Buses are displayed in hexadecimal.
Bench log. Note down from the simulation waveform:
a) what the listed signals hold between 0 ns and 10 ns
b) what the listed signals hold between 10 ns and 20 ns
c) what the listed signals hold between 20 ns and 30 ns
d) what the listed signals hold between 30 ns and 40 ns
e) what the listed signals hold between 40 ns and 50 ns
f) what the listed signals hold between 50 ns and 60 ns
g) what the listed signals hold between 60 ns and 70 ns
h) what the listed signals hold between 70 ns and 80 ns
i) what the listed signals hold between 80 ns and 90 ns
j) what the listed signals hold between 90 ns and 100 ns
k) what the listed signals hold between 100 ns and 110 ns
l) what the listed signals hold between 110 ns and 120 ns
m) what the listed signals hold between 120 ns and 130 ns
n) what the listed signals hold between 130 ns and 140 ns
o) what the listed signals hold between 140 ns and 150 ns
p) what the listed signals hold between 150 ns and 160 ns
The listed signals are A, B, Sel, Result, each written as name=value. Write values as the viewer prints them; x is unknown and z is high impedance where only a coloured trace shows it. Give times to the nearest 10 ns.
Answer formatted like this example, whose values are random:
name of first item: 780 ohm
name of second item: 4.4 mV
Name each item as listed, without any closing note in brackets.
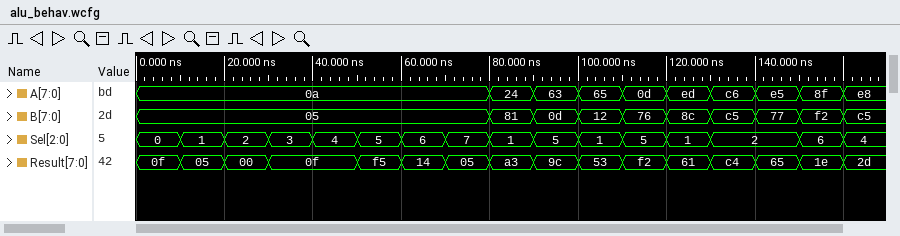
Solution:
what the listed signals hold between 0 ns and 10 ns: A=0a, B=05, Sel=0, Result=0f
what the listed signals hold between 10 ns and 20 ns: A=0a, B=05, Sel=1, Result=05
what the listed signals hold between 20 ns and 30 ns: A=0a, B=05, Sel=2, Result=00
what the listed signals hold between 30 ns and 40 ns: A=0a, B=05, Sel=3, Result=0f
what the listed signals hold between 40 ns and 50 ns: A=0a, B=05, Sel=4, Result=0f
what the listed signals hold between 50 ns and 60 ns: A=0a, B=05, Sel=5, Result=f5
what the listed signals hold between 60 ns and 70 ns: A=0a, B=05, Sel=6, Result=14
what the listed signals hold between 70 ns and 80 ns: A=0a, B=05, Sel=7, Result=05
what the listed signals hold between 80 ns and 90 ns: A=24, B=81, Sel=1, Result=a3
what the listed signals hold between 90 ns and 100 ns: A=63, B=0d, Sel=5, Result=9c
what the listed signals hold between 100 ns and 110 ns: A=65, B=12, Sel=1, Result=53
what the listed signals hold between 110 ns and 120 ns: A=0d, B=76, Sel=5, Result=f2
what the listed signals hold between 120 ns and 130 ns: A=ed, B=8c, Sel=1, Result=61
what the listed signals hold between 130 ns and 140 ns: A=c6, B=c5, Sel=2, Result=c4
what the listed signals hold between 140 ns and 150 ns: A=e5, B=77, Sel=2, Result=65
what the listed signals hold between 150 ns and 160 ns: A=8f, B=f2, Sel=6, Result=1e
